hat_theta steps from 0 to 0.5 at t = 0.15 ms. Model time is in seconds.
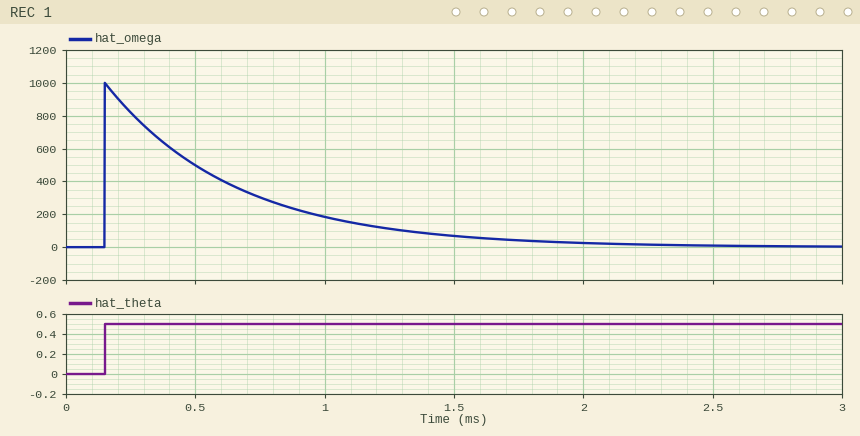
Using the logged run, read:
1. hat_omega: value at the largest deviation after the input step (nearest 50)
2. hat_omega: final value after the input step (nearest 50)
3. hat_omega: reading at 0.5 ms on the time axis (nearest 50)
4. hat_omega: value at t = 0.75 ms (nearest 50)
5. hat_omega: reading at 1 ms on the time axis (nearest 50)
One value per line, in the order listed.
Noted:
1000
0
500
300
200
